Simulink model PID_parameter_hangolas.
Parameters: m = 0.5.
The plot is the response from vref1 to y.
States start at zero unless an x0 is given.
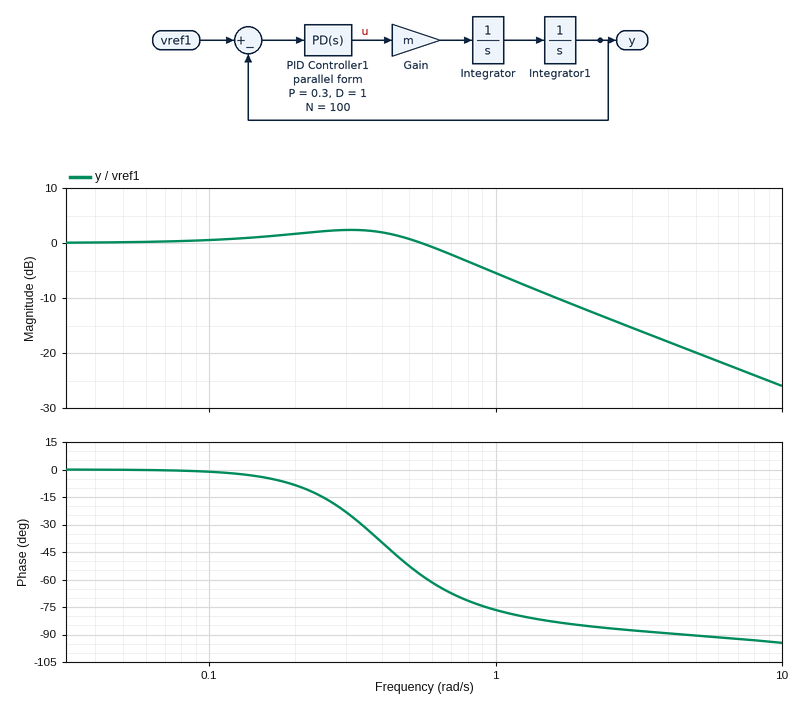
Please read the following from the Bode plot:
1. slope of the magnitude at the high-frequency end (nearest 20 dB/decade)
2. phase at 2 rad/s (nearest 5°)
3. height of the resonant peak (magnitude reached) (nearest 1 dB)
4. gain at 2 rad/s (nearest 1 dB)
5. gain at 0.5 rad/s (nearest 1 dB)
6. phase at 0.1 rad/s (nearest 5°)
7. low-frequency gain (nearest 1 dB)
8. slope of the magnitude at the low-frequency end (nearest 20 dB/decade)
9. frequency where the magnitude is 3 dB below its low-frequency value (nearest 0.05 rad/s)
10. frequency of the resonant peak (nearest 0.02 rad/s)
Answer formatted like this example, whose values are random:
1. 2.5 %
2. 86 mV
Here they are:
1. -20 dB/decade
2. -85°
3. 2 dB
4. -12 dB
5. 1 dB
6. 0°
7. 0 dB
8. 0 dB/decade
9. 0.75 rad/s
10. 0.30 rad/s
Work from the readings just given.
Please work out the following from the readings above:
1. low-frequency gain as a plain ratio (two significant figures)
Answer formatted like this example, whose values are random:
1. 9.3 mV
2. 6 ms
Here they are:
1. 1.0
